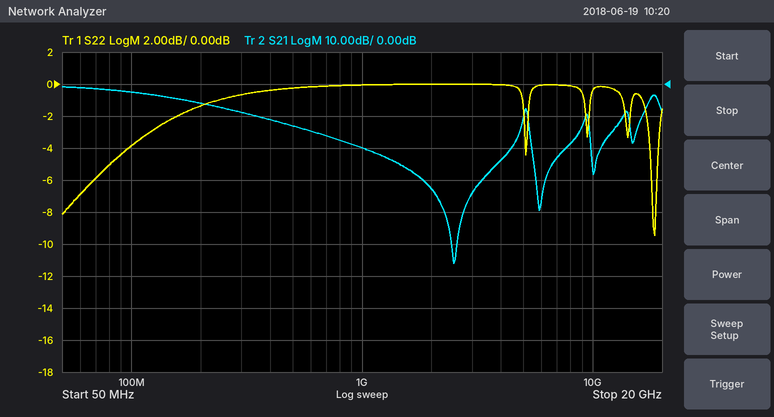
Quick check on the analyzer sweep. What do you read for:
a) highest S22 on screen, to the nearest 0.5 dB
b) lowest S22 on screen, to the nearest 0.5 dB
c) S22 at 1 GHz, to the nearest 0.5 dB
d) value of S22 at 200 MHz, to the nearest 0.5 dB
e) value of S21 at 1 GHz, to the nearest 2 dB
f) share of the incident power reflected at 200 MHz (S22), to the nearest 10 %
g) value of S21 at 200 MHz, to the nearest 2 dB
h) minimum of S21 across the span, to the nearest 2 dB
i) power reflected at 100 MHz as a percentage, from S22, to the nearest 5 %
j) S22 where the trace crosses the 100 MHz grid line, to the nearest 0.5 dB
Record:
0.0 dB
-9.5 dB
0.0 dB
-1.5 dB
-20 dB
70 %
-6 dB
-56 dB
40 %
-4.0 dB
